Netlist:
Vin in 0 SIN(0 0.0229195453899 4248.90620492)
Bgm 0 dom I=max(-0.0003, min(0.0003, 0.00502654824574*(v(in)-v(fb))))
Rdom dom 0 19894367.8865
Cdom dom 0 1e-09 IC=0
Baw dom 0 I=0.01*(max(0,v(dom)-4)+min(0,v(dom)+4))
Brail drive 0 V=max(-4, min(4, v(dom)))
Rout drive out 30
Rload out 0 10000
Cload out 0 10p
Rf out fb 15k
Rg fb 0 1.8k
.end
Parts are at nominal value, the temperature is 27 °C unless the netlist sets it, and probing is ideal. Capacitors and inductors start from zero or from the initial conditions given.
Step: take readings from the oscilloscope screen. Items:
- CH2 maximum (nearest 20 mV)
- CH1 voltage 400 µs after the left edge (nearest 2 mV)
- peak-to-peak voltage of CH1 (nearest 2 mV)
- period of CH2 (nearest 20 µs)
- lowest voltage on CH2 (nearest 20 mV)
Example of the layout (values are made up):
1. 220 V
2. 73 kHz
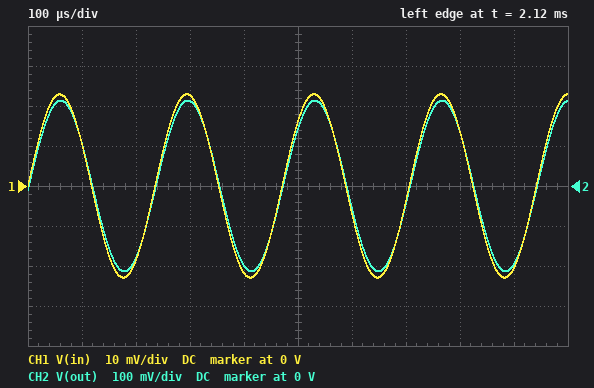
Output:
1. 220 mV
2. -22 mV
3. 46 mV
4. 240 µs
5. -220 mV
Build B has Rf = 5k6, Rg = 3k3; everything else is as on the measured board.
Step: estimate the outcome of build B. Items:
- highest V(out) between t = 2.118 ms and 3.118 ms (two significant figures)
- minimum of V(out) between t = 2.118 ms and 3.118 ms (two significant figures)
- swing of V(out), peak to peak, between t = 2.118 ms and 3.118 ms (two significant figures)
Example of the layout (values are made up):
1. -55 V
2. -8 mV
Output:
1. 62 mV
2. -62 mV
3. 120 mV
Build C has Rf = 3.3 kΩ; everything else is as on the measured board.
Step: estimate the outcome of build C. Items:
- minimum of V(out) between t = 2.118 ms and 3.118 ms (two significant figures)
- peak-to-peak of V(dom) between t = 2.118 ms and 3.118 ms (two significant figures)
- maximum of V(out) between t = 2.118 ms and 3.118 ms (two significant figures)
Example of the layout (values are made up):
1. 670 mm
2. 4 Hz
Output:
1. -65 mV
2. 130 mV
3. 65 mV
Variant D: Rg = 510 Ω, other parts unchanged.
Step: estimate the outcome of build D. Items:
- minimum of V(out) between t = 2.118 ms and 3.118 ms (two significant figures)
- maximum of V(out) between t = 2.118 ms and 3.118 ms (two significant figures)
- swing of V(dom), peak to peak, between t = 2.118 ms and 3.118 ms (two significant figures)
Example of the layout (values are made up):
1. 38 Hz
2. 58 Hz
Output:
1. -690 mV
2. 690 mV
3. 1.4 V
